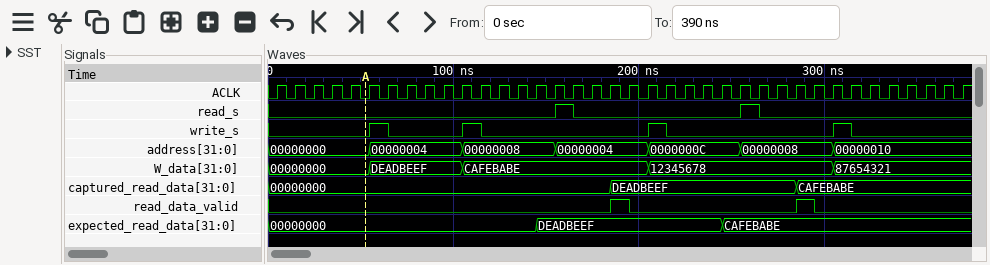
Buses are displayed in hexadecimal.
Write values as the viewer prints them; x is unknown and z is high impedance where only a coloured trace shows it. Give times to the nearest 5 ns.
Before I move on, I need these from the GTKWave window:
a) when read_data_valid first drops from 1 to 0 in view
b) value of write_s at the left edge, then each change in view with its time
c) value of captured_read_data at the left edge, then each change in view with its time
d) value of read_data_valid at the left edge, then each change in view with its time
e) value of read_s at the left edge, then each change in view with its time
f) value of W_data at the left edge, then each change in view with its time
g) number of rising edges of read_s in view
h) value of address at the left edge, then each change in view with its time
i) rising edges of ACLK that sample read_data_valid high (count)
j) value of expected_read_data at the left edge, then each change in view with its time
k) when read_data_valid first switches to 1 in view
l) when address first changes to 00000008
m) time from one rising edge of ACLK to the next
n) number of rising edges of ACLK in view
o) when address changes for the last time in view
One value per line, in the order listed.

195 ns
0, 1 at 55 ns, 0 at 65 ns, 1 at 105 ns, 0 at 115 ns, 1 at 205 ns, 0 at 215 ns, 1 at 305 ns, 0 at 315 ns
00000000, DEADBEEF at 185 ns, CAFEBABE at 285 ns
0, 1 at 185 ns, 0 at 195 ns, 1 at 285 ns, 0 at 295 ns
0, 1 at 155 ns, 0 at 165 ns, 1 at 255 ns, 0 at 265 ns
00000000, DEADBEEF at 55 ns, CAFEBABE at 105 ns, 12345678 at 205 ns, 87654321 at 305 ns
2
00000000, 00000004 at 55 ns, 00000008 at 105 ns, 00000004 at 155 ns, 0000000C at 205 ns, 00000008 at 255 ns, 00000010 at 305 ns
2
00000000, DEADBEEF at 145 ns, CAFEBABE at 245 ns
185 ns
105 ns
10 ns
38
305 ns
